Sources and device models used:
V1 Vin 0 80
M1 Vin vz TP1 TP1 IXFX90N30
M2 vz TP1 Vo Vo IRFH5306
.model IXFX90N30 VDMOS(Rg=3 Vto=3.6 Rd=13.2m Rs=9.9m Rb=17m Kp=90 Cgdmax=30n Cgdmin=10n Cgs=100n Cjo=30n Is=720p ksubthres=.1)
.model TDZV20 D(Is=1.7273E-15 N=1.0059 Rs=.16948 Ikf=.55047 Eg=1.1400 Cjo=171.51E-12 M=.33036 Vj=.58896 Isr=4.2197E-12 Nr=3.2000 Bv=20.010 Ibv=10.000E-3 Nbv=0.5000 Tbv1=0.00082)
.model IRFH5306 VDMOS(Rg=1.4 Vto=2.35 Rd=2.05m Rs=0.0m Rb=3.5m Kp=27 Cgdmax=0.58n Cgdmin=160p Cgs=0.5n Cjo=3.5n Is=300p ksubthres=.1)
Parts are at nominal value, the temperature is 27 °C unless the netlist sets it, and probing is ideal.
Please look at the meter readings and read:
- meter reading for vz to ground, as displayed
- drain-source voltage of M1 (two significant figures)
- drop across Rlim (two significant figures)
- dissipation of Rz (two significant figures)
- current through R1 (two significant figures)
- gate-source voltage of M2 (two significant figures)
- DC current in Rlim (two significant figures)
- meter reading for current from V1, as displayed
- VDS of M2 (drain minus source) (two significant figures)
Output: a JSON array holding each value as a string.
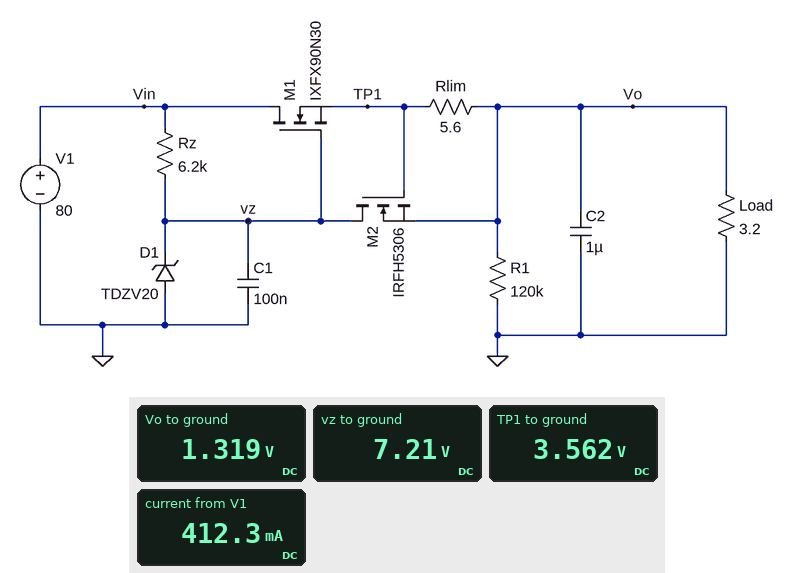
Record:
["7.21 V", "76 V", "2.2 V", "850 mW", "11 µA", "2.2 V", "400 mA", "412.3 mA", "5.9 V"]
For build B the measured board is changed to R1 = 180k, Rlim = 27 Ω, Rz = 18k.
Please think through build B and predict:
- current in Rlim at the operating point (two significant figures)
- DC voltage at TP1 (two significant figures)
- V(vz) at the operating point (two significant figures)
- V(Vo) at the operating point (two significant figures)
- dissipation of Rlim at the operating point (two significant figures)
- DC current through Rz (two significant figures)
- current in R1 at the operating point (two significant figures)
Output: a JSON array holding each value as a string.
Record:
["81 mA", "2.5 V", "6.0 V", "270 mV", "180 mW", "4.1 mA", "1.5 µA"]
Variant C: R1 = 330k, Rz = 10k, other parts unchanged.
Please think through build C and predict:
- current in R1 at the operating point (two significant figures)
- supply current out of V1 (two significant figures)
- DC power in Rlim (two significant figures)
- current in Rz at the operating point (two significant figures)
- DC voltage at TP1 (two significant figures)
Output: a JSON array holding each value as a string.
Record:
["3.9 µA", "400 mA", "880 mW", "7.3 mA", "3.5 V"]
